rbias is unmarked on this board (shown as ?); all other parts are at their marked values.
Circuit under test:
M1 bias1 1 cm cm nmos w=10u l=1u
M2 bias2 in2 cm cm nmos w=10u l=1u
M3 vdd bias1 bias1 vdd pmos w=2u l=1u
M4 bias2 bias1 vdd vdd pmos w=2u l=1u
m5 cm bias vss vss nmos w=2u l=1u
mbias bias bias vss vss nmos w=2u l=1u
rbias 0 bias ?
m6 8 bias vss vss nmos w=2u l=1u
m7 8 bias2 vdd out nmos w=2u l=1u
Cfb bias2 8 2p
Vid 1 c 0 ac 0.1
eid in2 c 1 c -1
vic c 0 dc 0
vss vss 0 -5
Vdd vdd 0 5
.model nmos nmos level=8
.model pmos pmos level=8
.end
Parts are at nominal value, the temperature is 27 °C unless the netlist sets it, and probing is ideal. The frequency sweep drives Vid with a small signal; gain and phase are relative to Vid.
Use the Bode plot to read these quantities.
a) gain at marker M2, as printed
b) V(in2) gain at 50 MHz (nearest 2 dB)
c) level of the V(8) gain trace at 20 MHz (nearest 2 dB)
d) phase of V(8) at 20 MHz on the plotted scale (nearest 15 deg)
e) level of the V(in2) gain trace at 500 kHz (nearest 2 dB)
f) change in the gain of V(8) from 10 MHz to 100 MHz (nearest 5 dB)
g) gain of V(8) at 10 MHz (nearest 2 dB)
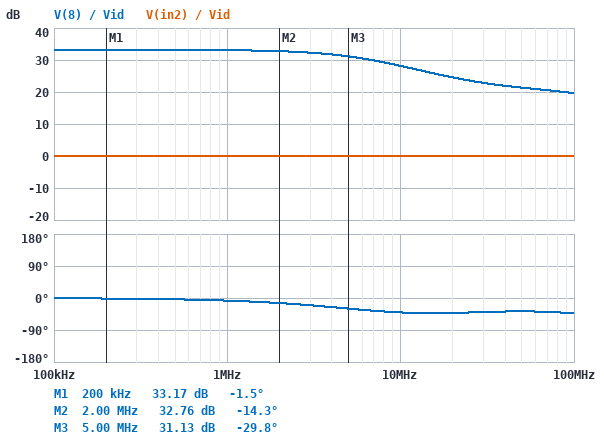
32.76 dB
0 dB
24 dB
-45 deg
0 dB
-10 dB
28 dB
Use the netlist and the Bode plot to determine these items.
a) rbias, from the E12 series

390 kΩ
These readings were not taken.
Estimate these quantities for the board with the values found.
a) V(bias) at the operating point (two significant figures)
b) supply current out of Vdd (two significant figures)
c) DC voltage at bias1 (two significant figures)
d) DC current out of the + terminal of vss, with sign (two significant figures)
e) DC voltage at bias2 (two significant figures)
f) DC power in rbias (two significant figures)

-4.6 V
360 µA
4.4 V
-370 µA
4.4 V
55 µW
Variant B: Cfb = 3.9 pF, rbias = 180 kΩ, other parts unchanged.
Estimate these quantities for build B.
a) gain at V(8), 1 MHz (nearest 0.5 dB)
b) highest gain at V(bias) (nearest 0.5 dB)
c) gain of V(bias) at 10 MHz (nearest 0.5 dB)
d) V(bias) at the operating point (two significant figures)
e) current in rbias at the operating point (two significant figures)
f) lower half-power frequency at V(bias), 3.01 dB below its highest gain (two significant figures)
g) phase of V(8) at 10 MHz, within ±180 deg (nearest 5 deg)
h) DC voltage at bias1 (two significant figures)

31.0 dB
-19.5 dB
-41.0 dB
-4.6 V
25 µA
200 MHz
-45 deg
4.3 V
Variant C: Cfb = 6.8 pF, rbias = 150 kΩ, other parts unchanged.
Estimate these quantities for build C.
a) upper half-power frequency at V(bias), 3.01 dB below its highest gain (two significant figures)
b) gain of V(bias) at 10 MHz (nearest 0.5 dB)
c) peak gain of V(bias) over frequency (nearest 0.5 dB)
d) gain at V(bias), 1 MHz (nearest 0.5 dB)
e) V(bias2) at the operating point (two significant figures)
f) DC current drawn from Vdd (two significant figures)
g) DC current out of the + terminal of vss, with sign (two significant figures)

2.2 GHz
-44.5 dB
-19.5 dB
-54.5 dB
4.2 V
620 µA
-650 µA
